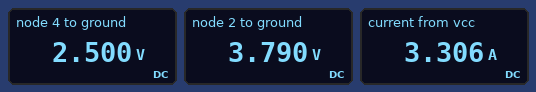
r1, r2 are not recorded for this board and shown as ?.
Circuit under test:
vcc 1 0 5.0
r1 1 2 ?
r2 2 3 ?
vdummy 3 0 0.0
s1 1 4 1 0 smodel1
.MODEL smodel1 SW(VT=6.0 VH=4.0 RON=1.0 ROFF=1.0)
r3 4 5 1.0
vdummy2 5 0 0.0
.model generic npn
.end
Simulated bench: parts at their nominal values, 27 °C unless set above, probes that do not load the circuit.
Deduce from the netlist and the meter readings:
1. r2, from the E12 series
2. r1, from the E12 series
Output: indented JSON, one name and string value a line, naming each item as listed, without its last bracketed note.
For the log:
{
  "r2, from the E12 series": "4.7 Ω",
  "r1, from the E12 series": "1.5 Ω"
}
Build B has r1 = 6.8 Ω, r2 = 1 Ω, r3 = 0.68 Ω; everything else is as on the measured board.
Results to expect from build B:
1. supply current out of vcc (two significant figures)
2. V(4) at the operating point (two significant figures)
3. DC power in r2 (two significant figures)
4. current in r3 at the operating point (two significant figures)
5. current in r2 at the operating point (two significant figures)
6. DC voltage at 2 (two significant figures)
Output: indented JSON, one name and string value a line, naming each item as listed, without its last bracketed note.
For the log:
{
  "supply current out of vcc": "3.6 A",
  "V(4) at the operating point": "2.0 V",
  "DC power in r2": "410 mW",
  "current in r3 at the operating point": "3.0 A",
  "current in r2 at the operating point": "640 mA",
  "DC voltage at 2": "640 mV"
}
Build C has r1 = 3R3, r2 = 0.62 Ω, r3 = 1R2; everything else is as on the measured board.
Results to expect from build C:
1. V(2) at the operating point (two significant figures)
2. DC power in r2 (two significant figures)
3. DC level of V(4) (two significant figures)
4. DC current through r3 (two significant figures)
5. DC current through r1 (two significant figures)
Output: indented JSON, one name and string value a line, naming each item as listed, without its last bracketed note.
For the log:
{
  "V(2) at the operating point": "790 mV",
  "DC power in r2": "1.0 W",
  "DC level of V(4)": "2.7 V",
  "DC current through r3": "2.3 A",
  "DC current through r1": "1.3 A"
}
